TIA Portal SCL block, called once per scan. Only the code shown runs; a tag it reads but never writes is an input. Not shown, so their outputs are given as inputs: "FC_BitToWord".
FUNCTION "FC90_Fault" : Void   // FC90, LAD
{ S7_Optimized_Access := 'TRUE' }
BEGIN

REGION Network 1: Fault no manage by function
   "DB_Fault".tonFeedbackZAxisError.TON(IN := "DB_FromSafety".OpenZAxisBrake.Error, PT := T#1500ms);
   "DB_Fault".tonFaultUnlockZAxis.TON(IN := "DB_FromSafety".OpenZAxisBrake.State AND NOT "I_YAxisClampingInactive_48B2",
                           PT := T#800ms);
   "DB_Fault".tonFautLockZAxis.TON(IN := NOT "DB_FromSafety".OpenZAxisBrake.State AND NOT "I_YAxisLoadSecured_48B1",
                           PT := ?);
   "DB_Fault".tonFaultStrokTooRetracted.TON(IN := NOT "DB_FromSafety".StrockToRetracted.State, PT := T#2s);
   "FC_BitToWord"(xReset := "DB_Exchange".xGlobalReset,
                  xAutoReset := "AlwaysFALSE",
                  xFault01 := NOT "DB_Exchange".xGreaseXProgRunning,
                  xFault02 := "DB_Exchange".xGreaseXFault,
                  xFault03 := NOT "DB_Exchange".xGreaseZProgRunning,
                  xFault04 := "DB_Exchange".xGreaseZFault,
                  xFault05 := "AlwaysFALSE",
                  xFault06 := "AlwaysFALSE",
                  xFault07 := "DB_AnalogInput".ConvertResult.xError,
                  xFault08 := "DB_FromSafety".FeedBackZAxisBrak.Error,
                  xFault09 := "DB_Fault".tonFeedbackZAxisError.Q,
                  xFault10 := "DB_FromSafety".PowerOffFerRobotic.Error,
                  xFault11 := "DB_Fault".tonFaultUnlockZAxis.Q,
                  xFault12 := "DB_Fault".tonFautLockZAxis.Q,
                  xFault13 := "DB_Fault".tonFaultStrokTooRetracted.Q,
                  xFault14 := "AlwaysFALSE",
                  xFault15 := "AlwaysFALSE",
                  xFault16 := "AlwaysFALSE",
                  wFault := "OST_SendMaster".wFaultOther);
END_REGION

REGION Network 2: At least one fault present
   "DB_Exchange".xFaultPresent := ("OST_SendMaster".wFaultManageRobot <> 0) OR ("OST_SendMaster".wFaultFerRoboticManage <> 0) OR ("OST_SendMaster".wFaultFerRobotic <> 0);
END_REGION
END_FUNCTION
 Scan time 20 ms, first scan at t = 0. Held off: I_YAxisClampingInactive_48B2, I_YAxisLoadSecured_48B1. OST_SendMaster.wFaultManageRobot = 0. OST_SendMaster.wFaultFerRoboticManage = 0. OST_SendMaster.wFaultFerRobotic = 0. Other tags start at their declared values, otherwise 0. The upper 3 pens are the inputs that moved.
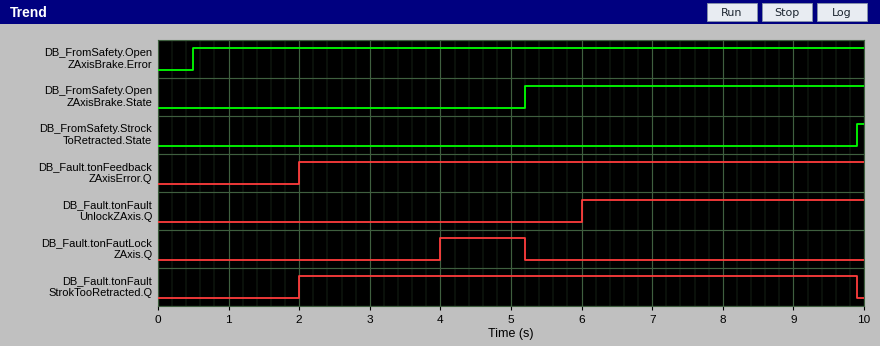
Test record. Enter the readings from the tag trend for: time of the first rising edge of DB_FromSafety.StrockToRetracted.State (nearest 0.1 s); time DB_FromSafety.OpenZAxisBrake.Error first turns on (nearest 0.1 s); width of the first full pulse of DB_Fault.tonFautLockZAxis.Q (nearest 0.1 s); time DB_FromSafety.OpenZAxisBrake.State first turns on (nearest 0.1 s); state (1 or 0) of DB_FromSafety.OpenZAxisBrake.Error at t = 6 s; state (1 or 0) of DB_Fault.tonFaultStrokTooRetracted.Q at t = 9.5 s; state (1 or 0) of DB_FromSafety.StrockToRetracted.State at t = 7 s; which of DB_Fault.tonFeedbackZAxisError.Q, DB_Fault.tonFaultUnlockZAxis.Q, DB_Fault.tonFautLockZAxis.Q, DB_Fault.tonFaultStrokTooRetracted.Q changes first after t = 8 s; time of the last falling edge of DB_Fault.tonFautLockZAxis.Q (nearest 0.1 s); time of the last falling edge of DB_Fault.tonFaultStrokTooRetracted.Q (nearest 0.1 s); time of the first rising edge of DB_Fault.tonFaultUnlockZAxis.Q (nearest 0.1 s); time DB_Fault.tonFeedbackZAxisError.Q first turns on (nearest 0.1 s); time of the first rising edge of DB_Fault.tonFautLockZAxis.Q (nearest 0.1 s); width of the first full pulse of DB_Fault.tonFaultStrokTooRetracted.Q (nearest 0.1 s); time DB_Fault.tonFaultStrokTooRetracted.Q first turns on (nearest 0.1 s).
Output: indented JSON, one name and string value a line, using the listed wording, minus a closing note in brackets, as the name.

{
  "time of the first rising edge of DB_FromSafety.StrockToRetracted.State": "9.9 s",
  "time DB_FromSafety.OpenZAxisBrake.Error first turns on": "0.5 s",
  "width of the first full pulse of DB_Fault.tonFautLockZAxis.Q": "1.2 s",
  "time DB_FromSafety.OpenZAxisBrake.State first turns on": "5.2 s",
  "state (1 or 0) of DB_FromSafety.OpenZAxisBrake.Error at t = 6 s": "1",
  "state (1 or 0) of DB_Fault.tonFaultStrokTooRetracted.Q at t = 9.5 s": "1",
  "state (1 or 0) of DB_FromSafety.StrockToRetracted.State at t = 7 s": "0",
  "which of DB_Fault.tonFeedbackZAxisError.Q, DB_Fault.tonFaultUnlockZAxis.Q, DB_Fault.tonFautLockZAxis.Q, DB_Fault.tonFaultStrokTooRetracted.Q changes first after t = 8 s": "DB_Fault.tonFaultStrokTooRetracted.Q",
  "time of the last falling edge of DB_Fault.tonFautLockZAxis.Q": "5.2 s",
  "time of the last falling edge of DB_Fault.tonFaultStrokTooRetracted.Q": "9.9 s",
  "time of the first rising edge of DB_Fault.tonFaultUnlockZAxis.Q": "6.0 s",
  "time DB_Fault.tonFeedbackZAxisError.Q first turns on": "2.0 s",
  "time of the first rising edge of DB_Fault.tonFautLockZAxis.Q": "4.0 s",
  "width of the first full pulse of DB_Fault.tonFaultStrokTooRetracted.Q": "7.9 s",
  "time DB_Fault.tonFaultStrokTooRetracted.Q first turns on": "2.0 s"
}
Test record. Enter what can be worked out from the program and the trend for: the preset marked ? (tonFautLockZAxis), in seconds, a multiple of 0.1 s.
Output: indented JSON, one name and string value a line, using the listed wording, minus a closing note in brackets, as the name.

{
  "the preset marked ? (tonFautLockZAxis), in seconds, a multiple of 0.1 s": "4.0 s"
}
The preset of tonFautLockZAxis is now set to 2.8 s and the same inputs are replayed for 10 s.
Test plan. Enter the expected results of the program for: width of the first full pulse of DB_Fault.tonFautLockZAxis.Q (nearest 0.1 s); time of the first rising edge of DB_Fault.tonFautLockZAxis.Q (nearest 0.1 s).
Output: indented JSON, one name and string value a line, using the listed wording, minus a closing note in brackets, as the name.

{
  "width of the first full pulse of DB_Fault.tonFautLockZAxis.Q": "2.4 s",
  "time of the first rising edge of DB_Fault.tonFautLockZAxis.Q": "2.8 s"
}
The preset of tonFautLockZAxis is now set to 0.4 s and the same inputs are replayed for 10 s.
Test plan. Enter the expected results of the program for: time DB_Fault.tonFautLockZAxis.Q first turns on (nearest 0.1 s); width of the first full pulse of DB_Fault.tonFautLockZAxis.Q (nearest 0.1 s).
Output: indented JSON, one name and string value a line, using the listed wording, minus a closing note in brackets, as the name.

{
  "time DB_Fault.tonFautLockZAxis.Q first turns on": "0.4 s",
  "width of the first full pulse of DB_Fault.tonFautLockZAxis.Q": "4.8 s"
}
